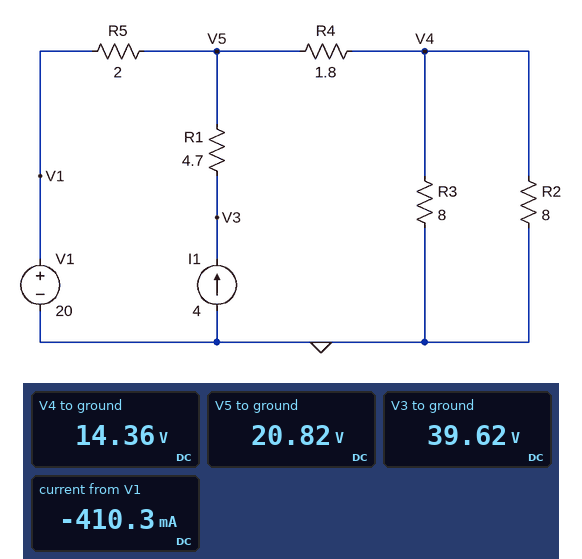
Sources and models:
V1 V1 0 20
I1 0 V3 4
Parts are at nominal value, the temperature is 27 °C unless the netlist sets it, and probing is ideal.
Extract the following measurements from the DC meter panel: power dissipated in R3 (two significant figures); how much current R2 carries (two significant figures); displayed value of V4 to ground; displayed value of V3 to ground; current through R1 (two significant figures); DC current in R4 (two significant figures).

26 W
1.8 A
14.36 V
39.62 V
4.0 A
3.6 A
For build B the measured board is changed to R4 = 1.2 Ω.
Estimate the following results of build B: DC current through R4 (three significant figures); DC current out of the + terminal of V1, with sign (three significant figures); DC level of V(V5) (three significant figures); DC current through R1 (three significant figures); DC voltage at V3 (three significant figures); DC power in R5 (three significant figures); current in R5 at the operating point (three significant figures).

3.89 A
-111 mA
20.2 V
4.00 A
39.0 V
24.7 mW
111 mA
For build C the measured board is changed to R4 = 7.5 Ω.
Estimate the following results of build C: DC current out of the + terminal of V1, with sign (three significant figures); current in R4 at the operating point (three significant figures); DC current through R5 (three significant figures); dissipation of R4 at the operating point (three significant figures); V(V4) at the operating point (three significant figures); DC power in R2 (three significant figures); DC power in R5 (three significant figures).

-1.93 A
2.07 A
1.93 A
32.3 W
8.30 V
8.60 W
7.42 W
